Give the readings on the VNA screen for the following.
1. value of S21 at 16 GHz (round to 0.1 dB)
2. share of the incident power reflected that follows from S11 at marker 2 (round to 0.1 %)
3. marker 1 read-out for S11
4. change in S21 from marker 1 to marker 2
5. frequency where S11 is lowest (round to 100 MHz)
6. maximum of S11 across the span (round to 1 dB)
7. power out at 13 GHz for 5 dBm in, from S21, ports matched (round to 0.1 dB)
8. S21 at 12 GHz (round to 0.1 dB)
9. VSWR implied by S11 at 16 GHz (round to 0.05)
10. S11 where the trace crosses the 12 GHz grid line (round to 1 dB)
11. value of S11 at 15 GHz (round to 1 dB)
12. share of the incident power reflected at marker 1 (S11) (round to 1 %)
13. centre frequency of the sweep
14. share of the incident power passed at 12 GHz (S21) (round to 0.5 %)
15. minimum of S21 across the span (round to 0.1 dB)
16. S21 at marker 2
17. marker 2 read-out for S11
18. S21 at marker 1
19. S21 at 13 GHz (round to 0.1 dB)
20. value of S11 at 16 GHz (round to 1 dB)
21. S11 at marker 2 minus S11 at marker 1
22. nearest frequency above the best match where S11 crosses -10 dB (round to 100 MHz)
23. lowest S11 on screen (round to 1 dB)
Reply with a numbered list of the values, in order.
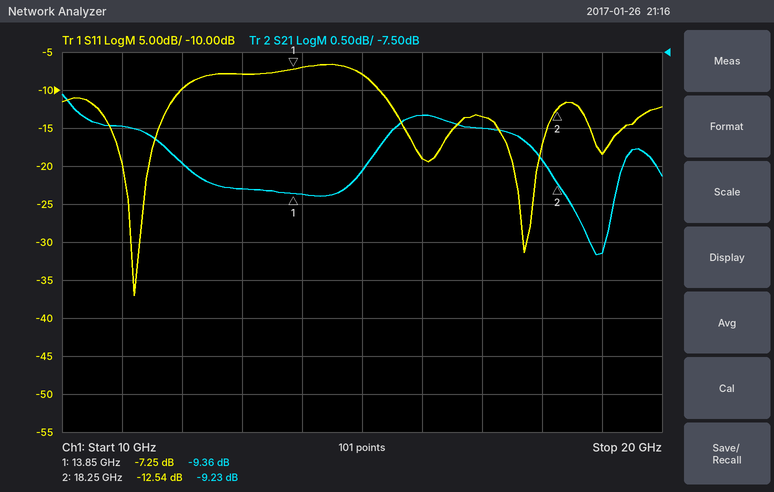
1. -8.3 dB
2. 5.6 %
3. -7.25 dB
4. 0.13 dB
5. 11.2 GHz
6. -7 dB
7. -4.3 dBm
8. -9.0 dB
9. 1.25
10. -10 dB
11. -8 dB
12. 19 %
13. 15 GHz
14. 12.5 %
15. -10.2 dB
16. -9.23 dB
17. -12.54 dB
18. -9.36 dB
19. -9.3 dB
20. -19 dB
21. -5.29 dB
22. 12.0 GHz
23. -37 dB
